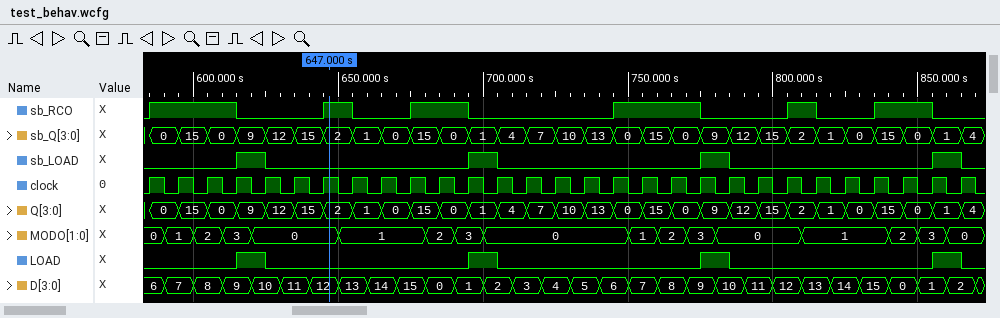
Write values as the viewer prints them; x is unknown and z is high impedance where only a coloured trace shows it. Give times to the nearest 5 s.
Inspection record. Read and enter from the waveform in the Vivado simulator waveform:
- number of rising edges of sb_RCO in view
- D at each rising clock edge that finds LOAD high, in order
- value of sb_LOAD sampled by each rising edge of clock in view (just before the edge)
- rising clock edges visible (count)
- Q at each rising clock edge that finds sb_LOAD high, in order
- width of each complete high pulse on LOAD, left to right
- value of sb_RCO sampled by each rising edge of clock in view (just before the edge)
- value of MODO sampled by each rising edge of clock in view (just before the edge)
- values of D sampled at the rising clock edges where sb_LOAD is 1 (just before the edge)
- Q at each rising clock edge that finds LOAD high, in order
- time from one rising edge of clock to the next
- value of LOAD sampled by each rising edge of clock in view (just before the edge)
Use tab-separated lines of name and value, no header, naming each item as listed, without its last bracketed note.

number of rising edges of sb_RCO in view	6
D at each rising clock edge that finds LOAD high, in order	10, 2, 10, 2
value of sb_LOAD sampled by each rising edge of clock in view	0 0 0 0 1 0 0 0 0 0 0 0 1 0 0 0 0 0 0 0 1 0 0 0 0 0 0 0 1
rising clock edges visible	29
Q at each rising clock edge that finds sb_LOAD high, in order	9, 1, 9, 1
width of each complete high pulse on LOAD, left to right	10 s, 10 s, 10 s, 10 s
value of sb_RCO sampled by each rising edge of clock in view	0 1 1 1 0 0 0 1 0 0 1 1 0 0 0 0 0 1 1 1 0 0 0 1 0 0 1 1 0
value of MODO sampled by each rising edge of clock in view	0, 1, 2, 3, 0, 0, 0, 1, 1, 1, 2, 3, 0, 0, 0, 0, 0, 1, 2, 3, 0, 0, 0, 1, 1, 1, 2, 3, 0
values of D sampled at the rising clock edges where sb_LOAD is 1	10, 2, 10, 2
Q at each rising clock edge that finds LOAD high, in order	9, 1, 9, 1
time from one rising edge of clock to the next	10 s
value of LOAD sampled by each rising edge of clock in view	0 0 0 0 1 0 0 0 0 0 0 0 1 0 0 0 0 0 0 0 1 0 0 0 0 0 0 0 1
